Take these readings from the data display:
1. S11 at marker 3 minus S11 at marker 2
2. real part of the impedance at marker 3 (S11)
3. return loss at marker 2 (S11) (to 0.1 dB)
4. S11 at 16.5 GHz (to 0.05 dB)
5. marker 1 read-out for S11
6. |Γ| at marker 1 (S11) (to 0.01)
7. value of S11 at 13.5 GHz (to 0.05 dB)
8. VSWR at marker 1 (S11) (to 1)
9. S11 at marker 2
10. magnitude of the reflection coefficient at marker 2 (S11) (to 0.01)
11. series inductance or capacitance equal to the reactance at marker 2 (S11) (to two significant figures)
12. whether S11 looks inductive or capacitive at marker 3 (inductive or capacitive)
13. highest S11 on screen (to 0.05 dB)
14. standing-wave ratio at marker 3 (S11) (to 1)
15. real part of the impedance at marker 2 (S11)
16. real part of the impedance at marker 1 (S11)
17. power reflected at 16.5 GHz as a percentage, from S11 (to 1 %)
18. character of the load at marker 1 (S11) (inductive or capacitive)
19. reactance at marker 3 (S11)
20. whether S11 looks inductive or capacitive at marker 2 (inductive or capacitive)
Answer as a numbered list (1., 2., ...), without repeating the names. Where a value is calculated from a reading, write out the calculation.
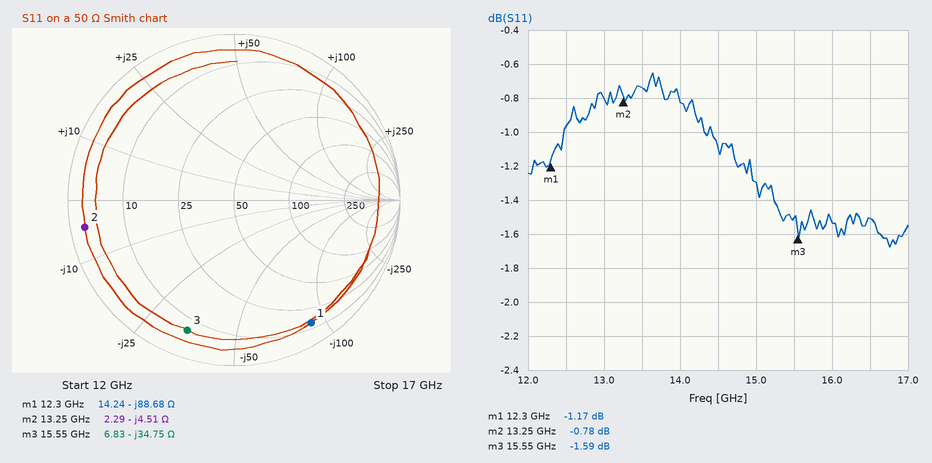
1. -1.59 − (-0.78) = -0.81 dB
2. 6.83 Ω
3. 0.8 dB
4. -1.50 dB
5. -1.17 dB
6. 0.87
7. -0.75 dB
8. (1 + 0.8740)/(1 − 0.8740) ≈ 15
9. -0.78 dB
10. 10^(-0.78/20) ≈ 0.91
11. C = 1/(2π × 13.25 GHz × 4.51 Ω) ≈ 2.7 pF
12. capacitive
13. -0.65 dB
14. 11
15. 2.29 Ω
16. 14.24 Ω
17. 10^(-1.5/10) ≈ 71 %
18. capacitive
19. -34.75 Ω
20. capacitive
